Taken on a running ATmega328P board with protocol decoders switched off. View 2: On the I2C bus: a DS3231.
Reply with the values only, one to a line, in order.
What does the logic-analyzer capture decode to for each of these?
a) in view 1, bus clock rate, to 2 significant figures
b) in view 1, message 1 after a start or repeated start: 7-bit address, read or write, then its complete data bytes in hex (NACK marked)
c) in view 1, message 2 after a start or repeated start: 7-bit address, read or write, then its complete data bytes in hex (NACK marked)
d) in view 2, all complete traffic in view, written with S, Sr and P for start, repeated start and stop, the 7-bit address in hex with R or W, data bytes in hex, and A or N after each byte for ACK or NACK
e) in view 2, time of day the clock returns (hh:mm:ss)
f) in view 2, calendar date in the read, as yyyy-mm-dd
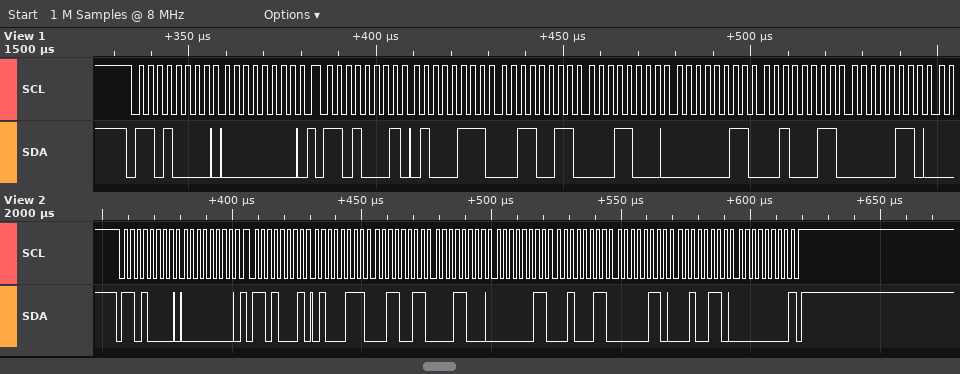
400 kHz
0x68 write: 00
0x68 read: 47 33 18 03 23 06
S 68W A 00 A Sr 68R A 47 A 33 A 18 A 03 A 23 A 06 A 26 A 00 N P
18:33:47
2026-06-23
